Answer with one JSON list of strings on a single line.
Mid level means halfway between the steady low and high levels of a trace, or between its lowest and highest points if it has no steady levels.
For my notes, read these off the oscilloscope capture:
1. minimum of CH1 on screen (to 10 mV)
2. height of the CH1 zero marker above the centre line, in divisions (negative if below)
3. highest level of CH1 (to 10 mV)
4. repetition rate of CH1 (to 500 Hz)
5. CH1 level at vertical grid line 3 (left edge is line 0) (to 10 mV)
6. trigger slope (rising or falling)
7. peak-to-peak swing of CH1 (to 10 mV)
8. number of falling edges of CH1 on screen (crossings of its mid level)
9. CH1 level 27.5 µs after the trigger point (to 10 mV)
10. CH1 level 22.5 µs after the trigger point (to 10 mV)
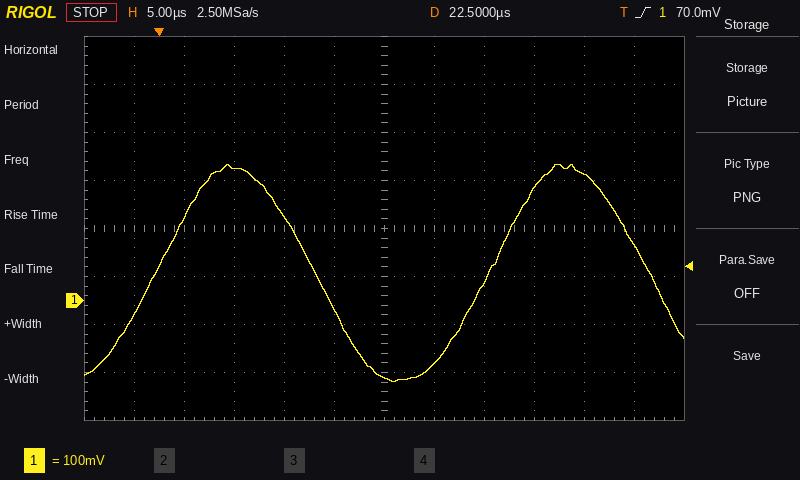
["-170 mV", "-1.5 div", "280 mV", "30.0 kHz", "280 mV", "rising", "450 mV", "2", "-130 mV", "-160 mV"]
